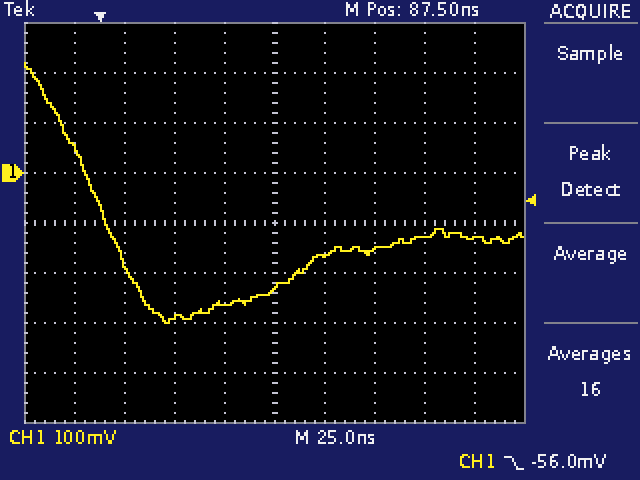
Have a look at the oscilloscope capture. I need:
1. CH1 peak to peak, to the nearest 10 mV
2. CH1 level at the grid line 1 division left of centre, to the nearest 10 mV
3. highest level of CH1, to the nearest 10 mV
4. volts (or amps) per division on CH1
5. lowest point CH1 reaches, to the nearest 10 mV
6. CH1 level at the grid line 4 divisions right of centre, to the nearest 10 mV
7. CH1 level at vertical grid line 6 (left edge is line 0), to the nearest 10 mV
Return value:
520 mV
-260 mV
220 mV
100 mV
-300 mV
-130 mV
-170 mV
